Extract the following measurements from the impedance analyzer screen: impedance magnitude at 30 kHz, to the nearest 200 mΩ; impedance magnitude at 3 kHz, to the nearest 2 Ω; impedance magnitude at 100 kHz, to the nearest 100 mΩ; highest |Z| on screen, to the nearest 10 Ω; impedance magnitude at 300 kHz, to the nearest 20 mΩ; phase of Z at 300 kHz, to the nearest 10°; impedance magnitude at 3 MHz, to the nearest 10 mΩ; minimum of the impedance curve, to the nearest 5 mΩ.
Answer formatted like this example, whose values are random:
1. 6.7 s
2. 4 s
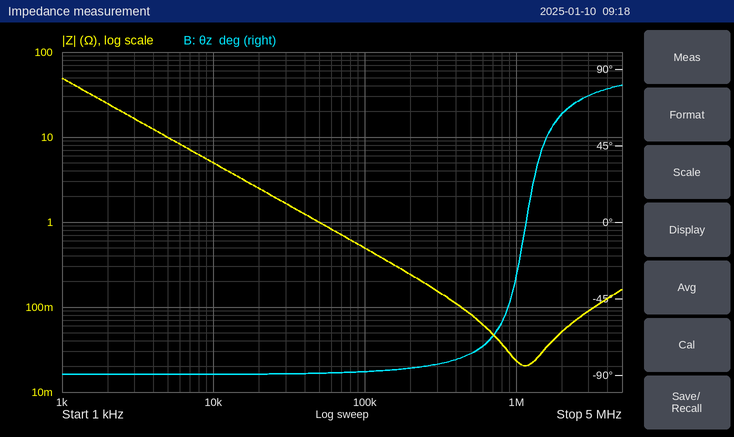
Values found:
1. 1.6 Ω
2. 16 Ω
3. 500 mΩ
4. 50 Ω
5. 160 mΩ
6. -80°
7. 90 mΩ
8. 20 mΩ
